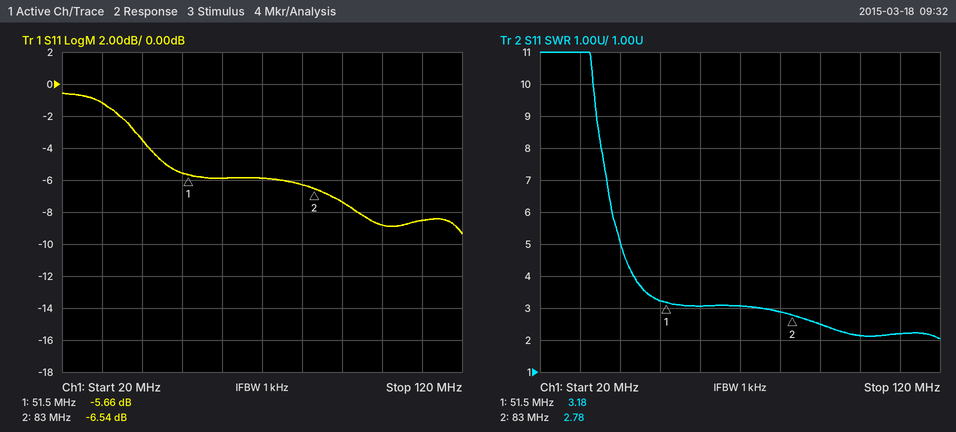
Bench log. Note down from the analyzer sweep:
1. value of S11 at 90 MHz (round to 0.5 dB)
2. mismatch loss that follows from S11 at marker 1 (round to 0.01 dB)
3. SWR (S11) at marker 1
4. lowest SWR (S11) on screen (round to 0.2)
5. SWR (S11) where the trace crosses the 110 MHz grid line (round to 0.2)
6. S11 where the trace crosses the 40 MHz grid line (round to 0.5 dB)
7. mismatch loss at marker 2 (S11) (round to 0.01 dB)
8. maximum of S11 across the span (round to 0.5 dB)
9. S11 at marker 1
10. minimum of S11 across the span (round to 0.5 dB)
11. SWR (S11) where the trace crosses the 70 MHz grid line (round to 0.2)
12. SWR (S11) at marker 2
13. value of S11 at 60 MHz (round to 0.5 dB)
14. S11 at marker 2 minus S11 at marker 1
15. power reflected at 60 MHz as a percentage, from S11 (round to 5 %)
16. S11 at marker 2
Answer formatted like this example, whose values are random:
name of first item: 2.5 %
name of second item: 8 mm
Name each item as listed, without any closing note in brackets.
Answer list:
value of S11 at 90 MHz: -7.5 dB
mismatch loss that follows from S11 at marker 1: 1.38 dB
SWR (S11) at marker 1: 3.18
lowest SWR (S11) on screen: 2.0
SWR (S11) where the trace crosses the 110 MHz grid line: 2.2
S11 where the trace crosses the 40 MHz grid line: -3.5 dB
mismatch loss at marker 2 (S11): 1.09 dB
maximum of S11 across the span: -0.5 dB
S11 at marker 1: -5.66 dB
minimum of S11 across the span: -9.5 dB
SWR (S11) where the trace crosses the 70 MHz grid line: 3.0
SWR (S11) at marker 2: 2.78
value of S11 at 60 MHz: -6.0 dB
S11 at marker 2 minus S11 at marker 1: -0.88 dB
power reflected at 60 MHz as a percentage, from S11: 25 %
S11 at marker 2: -6.54 dB
